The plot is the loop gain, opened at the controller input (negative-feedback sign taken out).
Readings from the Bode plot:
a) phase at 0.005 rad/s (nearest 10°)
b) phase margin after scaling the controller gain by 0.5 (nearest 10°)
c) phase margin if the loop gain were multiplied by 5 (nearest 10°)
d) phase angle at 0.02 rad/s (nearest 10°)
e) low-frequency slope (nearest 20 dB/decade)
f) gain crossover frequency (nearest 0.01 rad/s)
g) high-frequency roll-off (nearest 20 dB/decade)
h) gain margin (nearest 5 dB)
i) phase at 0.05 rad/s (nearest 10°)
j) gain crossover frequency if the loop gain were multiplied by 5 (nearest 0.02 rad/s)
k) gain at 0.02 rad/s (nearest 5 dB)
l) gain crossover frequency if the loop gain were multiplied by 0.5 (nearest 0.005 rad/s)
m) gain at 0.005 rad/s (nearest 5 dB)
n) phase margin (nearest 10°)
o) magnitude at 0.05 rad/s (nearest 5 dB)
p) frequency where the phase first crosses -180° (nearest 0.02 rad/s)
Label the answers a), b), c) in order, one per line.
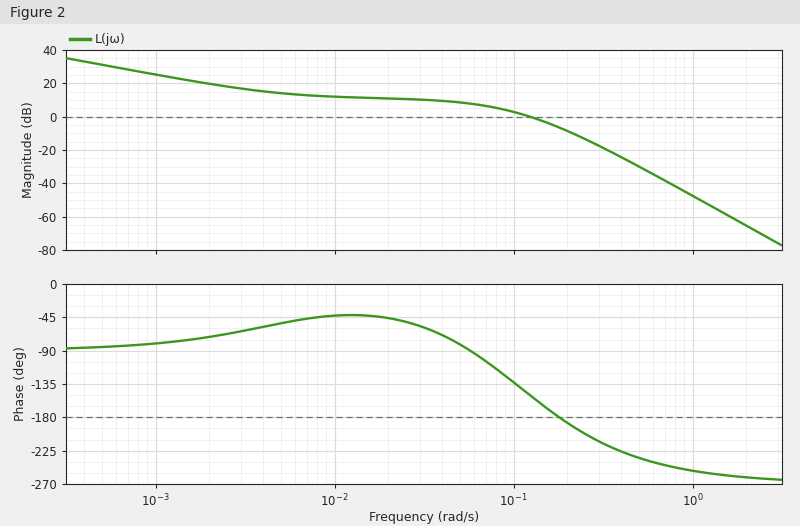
a) -50°
b) 70°
c) -20°
d) -50°
e) -20 dB/decade
f) 0.12 rad/s
g) -60 dB/decade
h) 5 dB
i) -80°
j) 0.26 rad/s
k) 10 dB
l) 0.075 rad/s
m) 15 dB
n) 30°
o) 10 dB
p) 0.18 rad/s
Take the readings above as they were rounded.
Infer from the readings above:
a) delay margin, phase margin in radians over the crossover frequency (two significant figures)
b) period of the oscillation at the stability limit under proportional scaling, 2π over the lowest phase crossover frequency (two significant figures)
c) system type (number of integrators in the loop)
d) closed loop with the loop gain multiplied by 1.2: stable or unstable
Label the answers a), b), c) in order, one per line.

a) 4.4 s
b) 35 s
c) 1
d) stable
